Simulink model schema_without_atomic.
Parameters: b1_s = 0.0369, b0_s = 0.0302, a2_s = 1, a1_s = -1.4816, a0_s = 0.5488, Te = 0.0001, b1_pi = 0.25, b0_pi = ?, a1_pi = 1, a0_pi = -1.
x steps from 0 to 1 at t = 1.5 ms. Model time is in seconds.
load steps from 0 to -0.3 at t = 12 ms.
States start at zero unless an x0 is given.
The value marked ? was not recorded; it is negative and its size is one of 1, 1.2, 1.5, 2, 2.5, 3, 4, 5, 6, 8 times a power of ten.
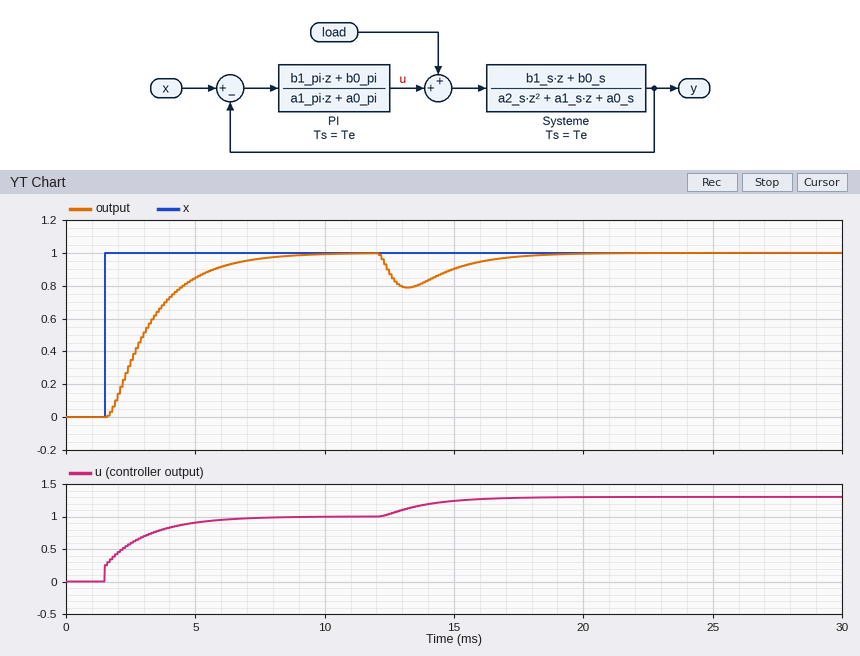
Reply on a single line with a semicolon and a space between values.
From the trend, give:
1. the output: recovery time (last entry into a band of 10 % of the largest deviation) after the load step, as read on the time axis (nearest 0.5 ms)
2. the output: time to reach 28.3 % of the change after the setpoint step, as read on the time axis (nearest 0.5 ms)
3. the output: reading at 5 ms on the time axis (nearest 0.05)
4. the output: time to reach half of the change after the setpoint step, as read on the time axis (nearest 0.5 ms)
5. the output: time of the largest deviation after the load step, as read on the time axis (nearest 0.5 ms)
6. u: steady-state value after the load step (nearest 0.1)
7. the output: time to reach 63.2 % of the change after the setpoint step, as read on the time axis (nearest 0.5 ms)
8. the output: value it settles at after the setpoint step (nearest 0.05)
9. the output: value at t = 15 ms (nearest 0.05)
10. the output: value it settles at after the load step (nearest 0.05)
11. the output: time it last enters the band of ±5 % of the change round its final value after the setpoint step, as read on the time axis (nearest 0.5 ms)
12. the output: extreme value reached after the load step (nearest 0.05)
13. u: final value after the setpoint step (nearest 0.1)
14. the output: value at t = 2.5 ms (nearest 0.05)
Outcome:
17.5 ms; 2.5 ms; 0.85; 3.0 ms; 13.0 ms; 1.3; 3.5 ms; 1.00; 0.90; 1.00; 7.0 ms; 0.80; 1.0; 0.35
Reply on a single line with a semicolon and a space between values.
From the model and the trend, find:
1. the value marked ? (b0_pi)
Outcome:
-0.2
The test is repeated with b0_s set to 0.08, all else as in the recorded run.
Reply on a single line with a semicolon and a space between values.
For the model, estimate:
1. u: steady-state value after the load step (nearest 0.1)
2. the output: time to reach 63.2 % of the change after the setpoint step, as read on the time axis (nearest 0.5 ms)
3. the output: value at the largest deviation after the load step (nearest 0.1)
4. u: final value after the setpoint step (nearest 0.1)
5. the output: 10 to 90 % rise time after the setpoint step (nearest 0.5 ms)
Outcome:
0.9; 2.5 ms; 0.7; 0.6; 2.0 ms
